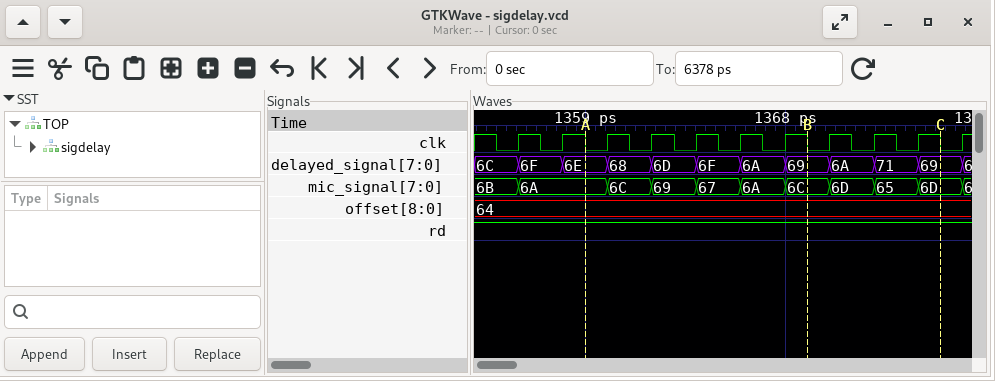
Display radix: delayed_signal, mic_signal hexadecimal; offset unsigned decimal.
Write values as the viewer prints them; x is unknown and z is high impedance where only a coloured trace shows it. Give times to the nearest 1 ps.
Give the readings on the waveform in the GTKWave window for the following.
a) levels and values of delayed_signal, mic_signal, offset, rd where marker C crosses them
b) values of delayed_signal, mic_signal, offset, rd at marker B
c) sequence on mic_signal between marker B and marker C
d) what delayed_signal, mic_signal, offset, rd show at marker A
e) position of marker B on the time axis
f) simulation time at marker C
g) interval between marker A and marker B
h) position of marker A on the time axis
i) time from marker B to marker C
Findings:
delayed_signal=69, mic_signal=6D, offset=64, rd=1
delayed_signal=69, mic_signal=6C, offset=64, rd=1
6C, 6D, 65, 6D
delayed_signal=6E, mic_signal=6A, offset=64, rd=1
1369 ps
1375 ps
10 ps
1359 ps
6 ps
